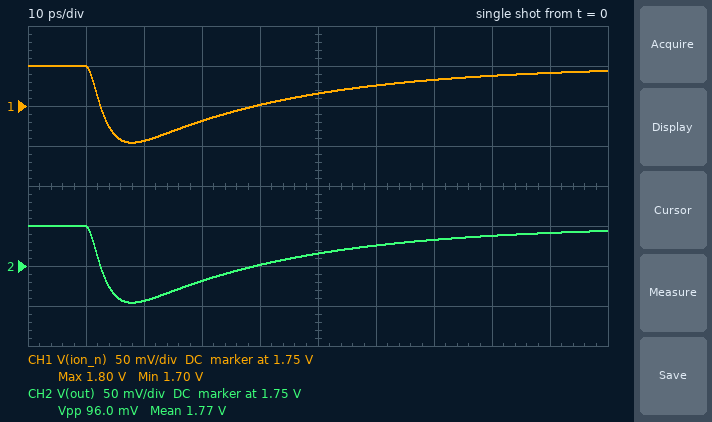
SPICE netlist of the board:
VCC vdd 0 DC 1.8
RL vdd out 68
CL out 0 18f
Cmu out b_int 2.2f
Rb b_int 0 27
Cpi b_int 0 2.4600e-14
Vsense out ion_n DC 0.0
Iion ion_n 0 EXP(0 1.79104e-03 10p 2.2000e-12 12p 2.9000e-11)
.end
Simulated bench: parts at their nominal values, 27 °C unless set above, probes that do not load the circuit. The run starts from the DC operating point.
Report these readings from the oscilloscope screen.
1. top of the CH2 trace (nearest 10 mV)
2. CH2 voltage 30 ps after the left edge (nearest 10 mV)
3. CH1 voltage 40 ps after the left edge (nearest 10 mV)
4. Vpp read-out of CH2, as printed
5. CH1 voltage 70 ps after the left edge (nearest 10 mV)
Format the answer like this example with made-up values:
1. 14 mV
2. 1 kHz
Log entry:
1. 1.80 V
2. 1.73 V
3. 1.75 V
4. 96.0 mV
5. 1.78 V
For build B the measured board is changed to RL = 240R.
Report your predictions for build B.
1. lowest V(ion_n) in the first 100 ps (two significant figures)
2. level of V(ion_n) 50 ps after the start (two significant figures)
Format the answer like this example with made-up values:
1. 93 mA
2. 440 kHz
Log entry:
1. 1.5 V
2. 1.7 V
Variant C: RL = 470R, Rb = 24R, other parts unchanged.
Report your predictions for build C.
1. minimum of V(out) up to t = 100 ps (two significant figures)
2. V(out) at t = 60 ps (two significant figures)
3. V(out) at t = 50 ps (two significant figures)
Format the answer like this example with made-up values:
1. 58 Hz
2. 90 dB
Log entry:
1. 1.3 V
2. 1.6 V
3. 1.5 V
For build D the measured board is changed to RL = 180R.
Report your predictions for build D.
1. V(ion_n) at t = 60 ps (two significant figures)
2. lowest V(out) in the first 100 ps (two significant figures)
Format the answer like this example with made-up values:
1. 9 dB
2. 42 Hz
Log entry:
1. 1.7 V
2. 1.6 V
